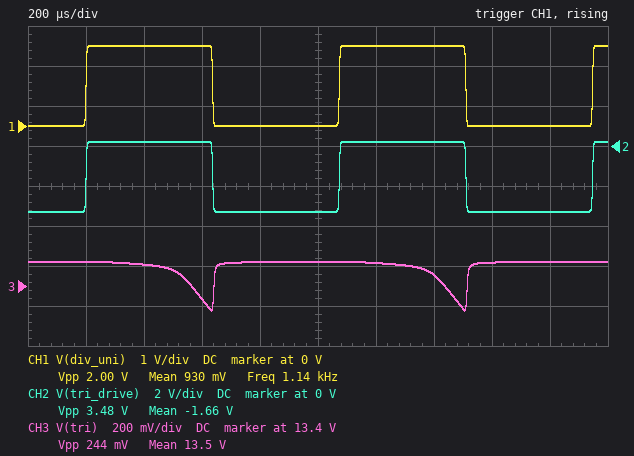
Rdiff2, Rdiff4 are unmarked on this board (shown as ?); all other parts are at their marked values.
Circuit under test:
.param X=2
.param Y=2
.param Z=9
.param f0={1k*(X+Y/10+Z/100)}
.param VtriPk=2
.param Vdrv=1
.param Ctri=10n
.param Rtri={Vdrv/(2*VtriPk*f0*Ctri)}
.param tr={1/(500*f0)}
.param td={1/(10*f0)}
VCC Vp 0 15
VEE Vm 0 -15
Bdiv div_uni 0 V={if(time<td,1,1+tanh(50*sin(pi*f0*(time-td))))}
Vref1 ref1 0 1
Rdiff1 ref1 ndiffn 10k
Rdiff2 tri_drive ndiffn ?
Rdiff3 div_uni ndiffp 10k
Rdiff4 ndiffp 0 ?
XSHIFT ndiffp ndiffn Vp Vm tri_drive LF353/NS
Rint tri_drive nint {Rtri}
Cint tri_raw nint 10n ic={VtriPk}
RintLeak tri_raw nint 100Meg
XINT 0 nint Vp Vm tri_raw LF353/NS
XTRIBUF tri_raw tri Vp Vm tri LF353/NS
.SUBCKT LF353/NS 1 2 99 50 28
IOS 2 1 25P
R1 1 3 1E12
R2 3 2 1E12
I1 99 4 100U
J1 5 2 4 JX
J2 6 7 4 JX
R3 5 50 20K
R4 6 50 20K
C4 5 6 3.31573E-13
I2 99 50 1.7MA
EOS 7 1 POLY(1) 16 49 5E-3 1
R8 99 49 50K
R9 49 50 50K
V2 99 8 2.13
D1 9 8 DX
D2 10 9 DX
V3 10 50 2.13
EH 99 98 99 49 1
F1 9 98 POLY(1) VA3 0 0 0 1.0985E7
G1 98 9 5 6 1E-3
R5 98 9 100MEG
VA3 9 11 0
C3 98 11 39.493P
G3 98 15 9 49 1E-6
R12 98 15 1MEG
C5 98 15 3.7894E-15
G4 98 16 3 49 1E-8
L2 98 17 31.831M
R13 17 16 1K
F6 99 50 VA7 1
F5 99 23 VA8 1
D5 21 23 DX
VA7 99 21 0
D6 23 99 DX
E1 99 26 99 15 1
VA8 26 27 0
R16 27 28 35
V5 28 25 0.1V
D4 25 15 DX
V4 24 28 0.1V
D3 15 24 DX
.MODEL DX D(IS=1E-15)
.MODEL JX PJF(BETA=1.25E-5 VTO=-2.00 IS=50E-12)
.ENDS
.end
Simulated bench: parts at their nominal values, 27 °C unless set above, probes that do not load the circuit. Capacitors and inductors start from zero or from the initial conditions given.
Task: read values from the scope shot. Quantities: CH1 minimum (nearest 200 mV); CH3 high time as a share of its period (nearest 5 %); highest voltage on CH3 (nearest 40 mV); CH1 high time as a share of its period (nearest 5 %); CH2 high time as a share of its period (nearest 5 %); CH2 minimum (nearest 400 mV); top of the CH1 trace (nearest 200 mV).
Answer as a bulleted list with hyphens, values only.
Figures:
- 0 V
- 90 %
- 13.52 V
- 50 %
- 50 %
- -3.2 V
- 2.0 V
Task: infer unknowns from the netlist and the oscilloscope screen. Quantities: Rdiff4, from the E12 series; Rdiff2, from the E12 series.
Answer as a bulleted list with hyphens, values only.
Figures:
- 6.8 kΩ
- 33 kΩ
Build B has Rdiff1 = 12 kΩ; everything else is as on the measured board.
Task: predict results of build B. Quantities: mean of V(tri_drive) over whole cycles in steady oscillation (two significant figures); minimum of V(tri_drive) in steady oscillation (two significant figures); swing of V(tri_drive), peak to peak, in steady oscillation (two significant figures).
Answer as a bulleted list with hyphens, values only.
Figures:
- -1.2 V
- -2.7 V
- 3.0 V
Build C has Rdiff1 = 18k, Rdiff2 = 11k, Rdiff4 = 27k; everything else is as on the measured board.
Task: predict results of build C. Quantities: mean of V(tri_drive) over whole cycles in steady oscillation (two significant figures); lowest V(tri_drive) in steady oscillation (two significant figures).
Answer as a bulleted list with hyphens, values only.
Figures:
- 570 mV
- -600 mV
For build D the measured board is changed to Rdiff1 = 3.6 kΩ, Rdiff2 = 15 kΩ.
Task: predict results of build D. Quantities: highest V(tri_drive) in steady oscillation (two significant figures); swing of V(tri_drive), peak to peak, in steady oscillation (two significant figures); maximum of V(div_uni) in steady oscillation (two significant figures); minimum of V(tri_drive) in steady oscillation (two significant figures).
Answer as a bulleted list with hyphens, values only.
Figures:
- 42 mV
- 4.2 V
- 2.0 V
- -4.1 V
